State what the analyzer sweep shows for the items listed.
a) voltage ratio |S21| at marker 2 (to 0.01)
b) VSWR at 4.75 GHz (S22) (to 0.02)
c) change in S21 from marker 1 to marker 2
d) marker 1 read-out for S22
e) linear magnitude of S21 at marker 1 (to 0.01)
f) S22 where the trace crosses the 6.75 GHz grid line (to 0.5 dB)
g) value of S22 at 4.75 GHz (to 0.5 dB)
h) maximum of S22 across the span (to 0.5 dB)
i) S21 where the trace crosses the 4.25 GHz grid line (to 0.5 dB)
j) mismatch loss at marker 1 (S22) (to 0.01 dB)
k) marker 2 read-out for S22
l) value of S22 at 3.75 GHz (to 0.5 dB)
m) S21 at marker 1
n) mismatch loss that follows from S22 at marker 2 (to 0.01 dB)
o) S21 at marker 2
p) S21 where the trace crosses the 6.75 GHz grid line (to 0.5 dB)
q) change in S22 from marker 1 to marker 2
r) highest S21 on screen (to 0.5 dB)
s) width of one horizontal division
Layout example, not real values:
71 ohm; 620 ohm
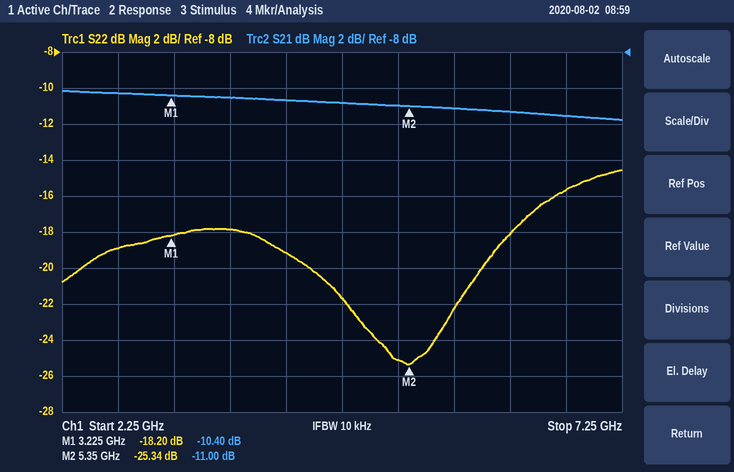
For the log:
0.28; 1.18; -0.60 dB; -18.20 dB; 0.30; -15.5 dB; -21.5 dB; -14.5 dB; -10.5 dB; 0.07 dB; -25.34 dB; -18.0 dB; -10.40 dB; 0.01 dB; -11.00 dB; -11.5 dB; -7.14 dB; -10.0 dB; 500 MHz
